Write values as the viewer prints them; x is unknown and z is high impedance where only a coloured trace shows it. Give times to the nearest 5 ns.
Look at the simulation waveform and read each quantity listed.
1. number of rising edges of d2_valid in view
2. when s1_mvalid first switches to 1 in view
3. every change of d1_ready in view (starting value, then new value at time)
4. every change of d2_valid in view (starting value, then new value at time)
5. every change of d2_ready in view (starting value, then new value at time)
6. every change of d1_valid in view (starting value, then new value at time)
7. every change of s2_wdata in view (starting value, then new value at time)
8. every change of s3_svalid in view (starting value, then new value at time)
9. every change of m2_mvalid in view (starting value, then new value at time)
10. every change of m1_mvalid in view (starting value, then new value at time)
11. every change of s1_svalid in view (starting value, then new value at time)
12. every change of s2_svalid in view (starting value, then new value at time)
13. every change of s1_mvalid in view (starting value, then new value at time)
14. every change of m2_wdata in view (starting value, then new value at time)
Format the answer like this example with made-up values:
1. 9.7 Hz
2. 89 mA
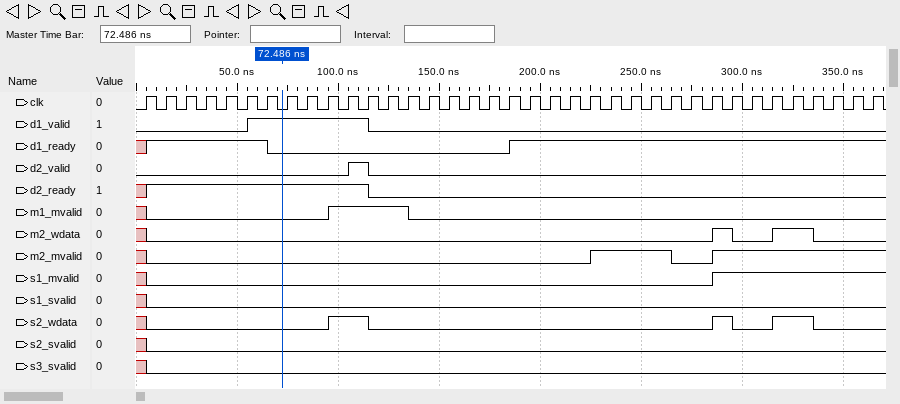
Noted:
1. 1
2. 285 ns
3. x, 1 at 5 ns, 0 at 65 ns, 1 at 185 ns
4. 0, 1 at 105 ns, 0 at 115 ns
5. x, 1 at 5 ns, 0 at 115 ns
6. 0, 1 at 55 ns, 0 at 115 ns
7. x, 0 at 5 ns, 1 at 95 ns, 0 at 115 ns, 1 at 285 ns, 0 at 295 ns, 1 at 315 ns, 0 at 335 ns
8. x, 0 at 5 ns
9. x, 0 at 5 ns, 1 at 225 ns, 0 at 265 ns, 1 at 285 ns
10. x, 0 at 5 ns, 1 at 95 ns, 0 at 135 ns
11. x, 0 at 5 ns
12. x, 0 at 5 ns
13. x, 0 at 5 ns, 1 at 285 ns
14. x, 0 at 5 ns, 1 at 285 ns, 0 at 295 ns, 1 at 315 ns, 0 at 335 ns
